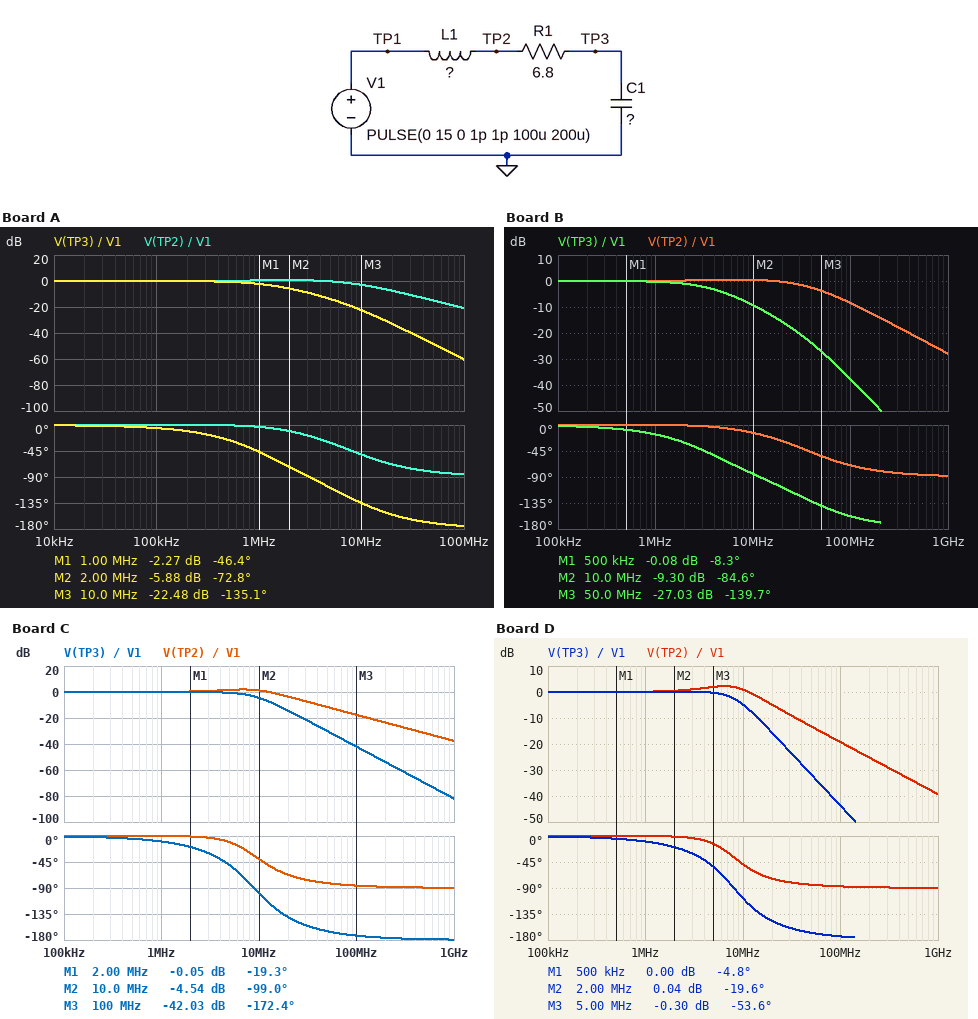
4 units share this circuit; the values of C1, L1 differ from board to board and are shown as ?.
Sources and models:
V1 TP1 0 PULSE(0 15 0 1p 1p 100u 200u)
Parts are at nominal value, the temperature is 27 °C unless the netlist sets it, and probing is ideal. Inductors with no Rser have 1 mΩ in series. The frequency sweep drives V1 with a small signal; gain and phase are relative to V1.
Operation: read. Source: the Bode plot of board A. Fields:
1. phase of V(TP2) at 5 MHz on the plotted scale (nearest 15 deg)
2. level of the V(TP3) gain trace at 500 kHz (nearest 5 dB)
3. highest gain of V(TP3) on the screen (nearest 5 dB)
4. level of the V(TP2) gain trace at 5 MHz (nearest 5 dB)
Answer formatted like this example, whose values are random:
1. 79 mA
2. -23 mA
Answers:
1. -30 deg
2. 0 dB
3. 0 dB
4. 0 dB
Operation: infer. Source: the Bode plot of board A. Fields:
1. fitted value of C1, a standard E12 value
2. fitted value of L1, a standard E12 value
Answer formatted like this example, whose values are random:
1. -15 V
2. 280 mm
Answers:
1. 22 nF
2. 120 nH
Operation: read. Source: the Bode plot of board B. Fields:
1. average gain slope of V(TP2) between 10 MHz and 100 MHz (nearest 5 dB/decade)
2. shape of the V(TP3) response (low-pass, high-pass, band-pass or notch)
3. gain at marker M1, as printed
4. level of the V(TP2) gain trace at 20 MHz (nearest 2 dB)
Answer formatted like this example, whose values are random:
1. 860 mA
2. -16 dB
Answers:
1. -10 dB/decade
2. low-pass
3. -0.08 dB
4. 0 dB
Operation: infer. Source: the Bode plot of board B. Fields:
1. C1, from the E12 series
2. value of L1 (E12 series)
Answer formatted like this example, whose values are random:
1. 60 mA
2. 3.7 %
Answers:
1. 6.8 nF
2. 27 nH
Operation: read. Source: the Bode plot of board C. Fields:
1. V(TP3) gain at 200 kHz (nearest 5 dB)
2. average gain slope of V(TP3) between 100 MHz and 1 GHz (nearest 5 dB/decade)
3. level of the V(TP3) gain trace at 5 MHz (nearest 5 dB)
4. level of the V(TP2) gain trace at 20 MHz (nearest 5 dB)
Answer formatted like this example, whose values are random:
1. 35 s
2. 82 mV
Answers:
1. 0 dB
2. -40 dB/decade
3. 0 dB
4. -5 dB
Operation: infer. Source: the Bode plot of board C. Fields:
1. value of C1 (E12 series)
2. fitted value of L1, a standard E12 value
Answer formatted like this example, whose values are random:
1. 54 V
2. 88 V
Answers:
1. 3.9 nF
2. 82 nH
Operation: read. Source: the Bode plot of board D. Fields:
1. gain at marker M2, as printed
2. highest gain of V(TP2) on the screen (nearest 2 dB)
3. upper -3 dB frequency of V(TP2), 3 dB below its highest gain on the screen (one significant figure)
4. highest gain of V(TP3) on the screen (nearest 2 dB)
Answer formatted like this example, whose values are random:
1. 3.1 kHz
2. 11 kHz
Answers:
1. 0.04 dB
2. 2 dB
3. 10 MHz
4. 0 dB
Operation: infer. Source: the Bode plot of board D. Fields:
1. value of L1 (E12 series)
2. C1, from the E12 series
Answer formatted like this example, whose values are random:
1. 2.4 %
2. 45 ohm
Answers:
1. 100 nH
2. 3.9 nF
